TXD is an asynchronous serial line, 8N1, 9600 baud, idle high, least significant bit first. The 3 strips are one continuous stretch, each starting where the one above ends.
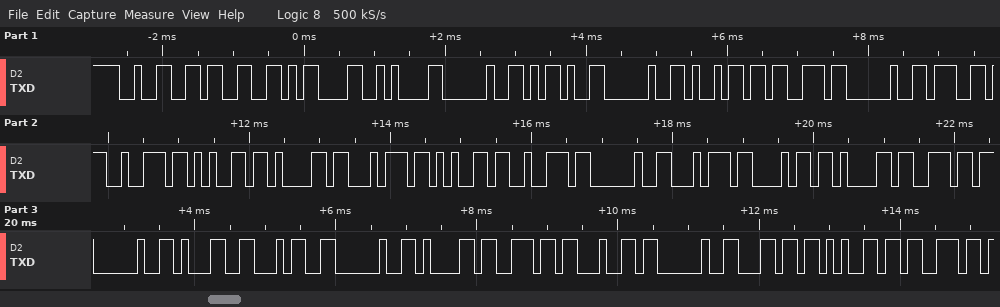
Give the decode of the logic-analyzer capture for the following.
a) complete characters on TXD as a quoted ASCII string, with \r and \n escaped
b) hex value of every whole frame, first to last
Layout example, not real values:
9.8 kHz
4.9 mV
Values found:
"23\r\n - is greater than 14 and les"
32 33 0D 0A 20 2D 20 69 73 20 67 72 65 61 74 65 72 20 74 68 61 6E 20 31 34 20 61 6E 64 20 6C 65 73
